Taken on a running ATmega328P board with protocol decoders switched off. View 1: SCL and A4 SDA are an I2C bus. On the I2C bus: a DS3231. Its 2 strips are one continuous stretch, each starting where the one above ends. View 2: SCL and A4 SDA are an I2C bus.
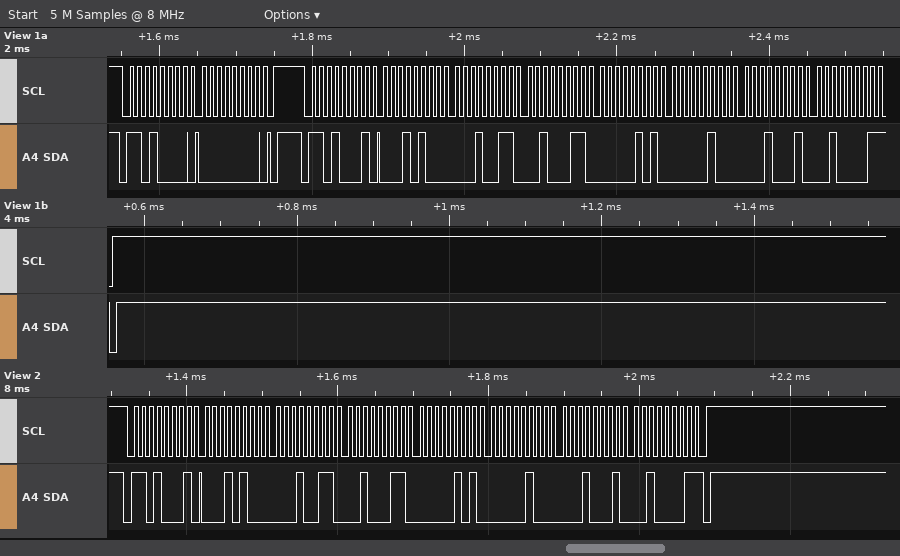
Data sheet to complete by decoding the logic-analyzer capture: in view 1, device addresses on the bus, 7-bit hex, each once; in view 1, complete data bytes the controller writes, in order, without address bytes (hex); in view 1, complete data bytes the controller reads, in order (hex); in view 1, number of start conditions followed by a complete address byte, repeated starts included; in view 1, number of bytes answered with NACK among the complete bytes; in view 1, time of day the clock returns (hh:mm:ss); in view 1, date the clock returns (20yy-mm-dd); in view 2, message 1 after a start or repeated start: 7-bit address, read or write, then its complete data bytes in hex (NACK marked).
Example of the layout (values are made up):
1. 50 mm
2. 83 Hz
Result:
1. 0x68
2. 00
3. 14 13 23 05 04 11 21
4. 2
5. 1
6. 23:13:14
7. 2021-11-04
8. 0x68 read: 14 13 23 05 04 11 21 NACK
